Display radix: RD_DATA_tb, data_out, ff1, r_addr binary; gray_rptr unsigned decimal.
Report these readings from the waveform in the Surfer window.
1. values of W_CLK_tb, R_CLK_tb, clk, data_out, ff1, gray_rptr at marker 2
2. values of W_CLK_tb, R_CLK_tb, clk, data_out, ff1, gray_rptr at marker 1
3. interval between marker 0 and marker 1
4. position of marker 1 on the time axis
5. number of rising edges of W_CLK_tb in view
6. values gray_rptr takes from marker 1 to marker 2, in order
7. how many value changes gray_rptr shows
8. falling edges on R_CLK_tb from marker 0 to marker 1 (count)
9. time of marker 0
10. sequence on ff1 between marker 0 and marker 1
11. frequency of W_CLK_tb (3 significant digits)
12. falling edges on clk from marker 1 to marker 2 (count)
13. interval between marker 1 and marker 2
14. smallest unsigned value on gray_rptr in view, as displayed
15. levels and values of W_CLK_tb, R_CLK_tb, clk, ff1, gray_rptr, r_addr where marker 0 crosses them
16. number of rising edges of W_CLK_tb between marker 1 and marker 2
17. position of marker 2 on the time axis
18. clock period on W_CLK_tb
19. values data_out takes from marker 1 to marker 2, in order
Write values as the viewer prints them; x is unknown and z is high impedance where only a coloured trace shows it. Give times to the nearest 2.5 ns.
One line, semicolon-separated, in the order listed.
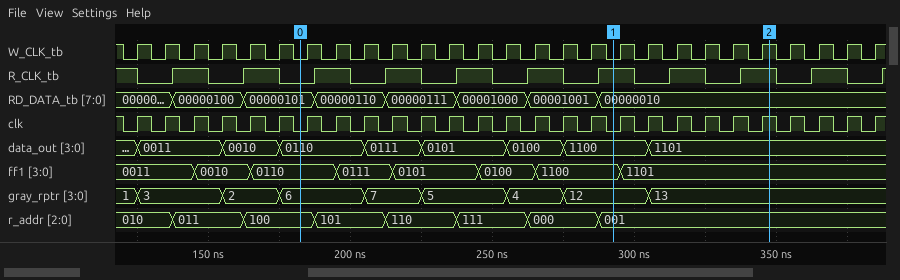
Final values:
W_CLK_tb=1, R_CLK_tb=1, clk=1, data_out=1101, ff1=1101, gray_rptr=13; W_CLK_tb=0, R_CLK_tb=1, clk=0, data_out=1100, ff1=1100, gray_rptr=12; 110 ns; 292.5 ns; 27; 12, 13; 8; 4; 182.5 ns; 0110, 0111, 0101, 0100, 1100; 100 MHz; 5; 55 ns; 1; W_CLK_tb=0, R_CLK_tb=0, clk=0, ff1=0110, gray_rptr=6, r_addr=100; 6; 347.5 ns; 10 ns; 1100, 1101
